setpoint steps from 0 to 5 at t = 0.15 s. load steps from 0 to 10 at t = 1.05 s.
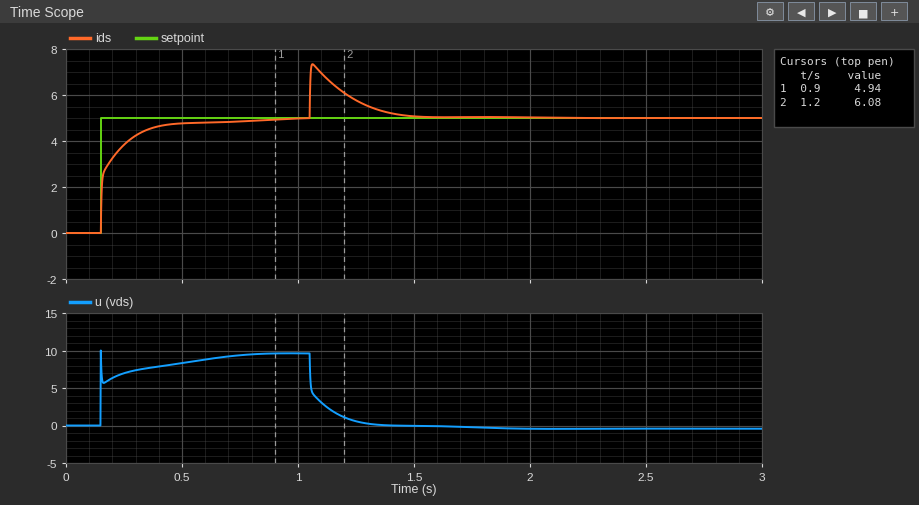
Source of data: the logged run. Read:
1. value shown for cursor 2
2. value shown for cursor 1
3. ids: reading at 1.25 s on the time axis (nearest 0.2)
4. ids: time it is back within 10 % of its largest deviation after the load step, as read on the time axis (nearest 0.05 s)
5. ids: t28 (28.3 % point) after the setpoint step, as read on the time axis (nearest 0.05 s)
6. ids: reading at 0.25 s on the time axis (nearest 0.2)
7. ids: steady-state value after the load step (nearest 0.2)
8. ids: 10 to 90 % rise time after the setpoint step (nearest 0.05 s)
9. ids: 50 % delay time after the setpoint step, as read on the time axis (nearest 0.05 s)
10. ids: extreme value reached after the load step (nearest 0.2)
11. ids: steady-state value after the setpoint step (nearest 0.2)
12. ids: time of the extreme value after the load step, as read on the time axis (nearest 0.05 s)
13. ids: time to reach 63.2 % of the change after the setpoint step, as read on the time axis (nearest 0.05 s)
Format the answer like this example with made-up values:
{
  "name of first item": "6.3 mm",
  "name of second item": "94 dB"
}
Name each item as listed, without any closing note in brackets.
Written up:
{
  "value shown for cursor 2": "6.08",
  "value shown for cursor 1": "4.94",
  "ids: reading at 1.25 s on the time axis": "5.8",
  "ids: time it is back within 10 % of its largest deviation after the load step, as read on the time axis": "1.40 s",
  "ids: t28 (28.3 % point) after the setpoint step, as read on the time axis": "0.15 s",
  "ids: reading at 0.25 s on the time axis": "3.8",
  "ids: steady-state value after the load step": "5.0",
  "ids: 10 to 90 % rise time after the setpoint step": "0.20 s",
  "ids: 50 % delay time after the setpoint step, as read on the time axis": "0.15 s",
  "ids: extreme value reached after the load step": "7.4",
  "ids: steady-state value after the setpoint step": "5.0",
  "ids: time of the extreme value after the load step, as read on the time axis": "1.05 s",
  "ids: time to reach 63.2 % of the change after the setpoint step, as read on the time axis": "0.20 s"
}
